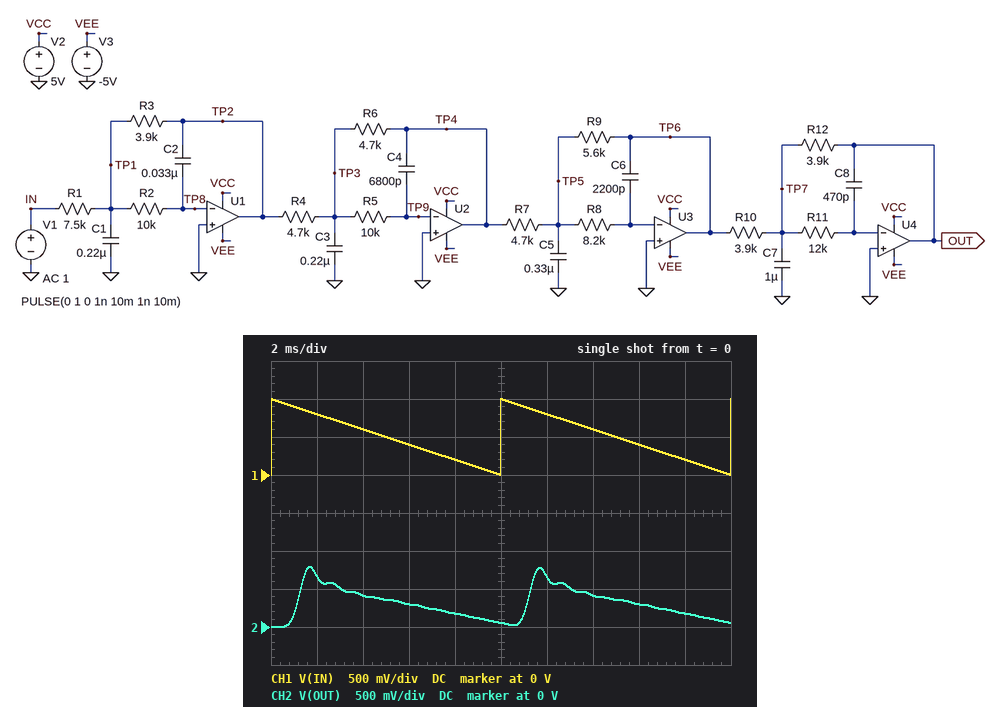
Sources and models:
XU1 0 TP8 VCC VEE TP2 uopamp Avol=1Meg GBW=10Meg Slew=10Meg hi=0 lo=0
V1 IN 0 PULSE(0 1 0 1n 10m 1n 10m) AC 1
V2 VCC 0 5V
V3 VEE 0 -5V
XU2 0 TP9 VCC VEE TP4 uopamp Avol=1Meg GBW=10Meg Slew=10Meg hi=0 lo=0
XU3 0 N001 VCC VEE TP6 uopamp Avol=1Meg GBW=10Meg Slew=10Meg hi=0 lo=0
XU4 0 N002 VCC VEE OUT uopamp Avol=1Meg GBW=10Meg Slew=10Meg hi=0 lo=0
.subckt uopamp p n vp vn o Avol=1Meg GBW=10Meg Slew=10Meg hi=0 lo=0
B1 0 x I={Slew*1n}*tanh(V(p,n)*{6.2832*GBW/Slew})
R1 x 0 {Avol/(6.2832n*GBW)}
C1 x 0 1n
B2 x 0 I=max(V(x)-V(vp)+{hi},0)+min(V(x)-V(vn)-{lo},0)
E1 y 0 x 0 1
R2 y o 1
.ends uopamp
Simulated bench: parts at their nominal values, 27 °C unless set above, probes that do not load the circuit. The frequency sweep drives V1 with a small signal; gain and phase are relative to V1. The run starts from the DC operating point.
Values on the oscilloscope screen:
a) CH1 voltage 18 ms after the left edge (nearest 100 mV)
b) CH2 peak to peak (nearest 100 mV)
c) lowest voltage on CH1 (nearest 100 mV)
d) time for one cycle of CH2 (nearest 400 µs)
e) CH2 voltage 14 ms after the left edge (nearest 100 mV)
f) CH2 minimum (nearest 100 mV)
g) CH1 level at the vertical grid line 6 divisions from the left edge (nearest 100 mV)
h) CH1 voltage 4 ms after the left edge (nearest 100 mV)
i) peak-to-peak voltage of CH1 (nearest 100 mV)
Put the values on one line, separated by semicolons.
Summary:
200 mV; 800 mV; 0 V; 10.0 ms; 400 mV; 0 V; 800 mV; 600 mV; 1.0 V
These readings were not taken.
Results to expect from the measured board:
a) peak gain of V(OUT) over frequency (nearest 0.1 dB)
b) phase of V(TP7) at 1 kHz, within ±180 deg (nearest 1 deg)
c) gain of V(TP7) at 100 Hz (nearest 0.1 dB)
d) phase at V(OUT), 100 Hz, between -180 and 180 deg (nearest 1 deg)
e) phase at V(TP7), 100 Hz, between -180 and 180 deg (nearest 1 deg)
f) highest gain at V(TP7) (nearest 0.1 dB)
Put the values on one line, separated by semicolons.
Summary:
-2.0 dB; 155 deg; -52.5 dB; -33 deg; -123 deg; -35.5 dB
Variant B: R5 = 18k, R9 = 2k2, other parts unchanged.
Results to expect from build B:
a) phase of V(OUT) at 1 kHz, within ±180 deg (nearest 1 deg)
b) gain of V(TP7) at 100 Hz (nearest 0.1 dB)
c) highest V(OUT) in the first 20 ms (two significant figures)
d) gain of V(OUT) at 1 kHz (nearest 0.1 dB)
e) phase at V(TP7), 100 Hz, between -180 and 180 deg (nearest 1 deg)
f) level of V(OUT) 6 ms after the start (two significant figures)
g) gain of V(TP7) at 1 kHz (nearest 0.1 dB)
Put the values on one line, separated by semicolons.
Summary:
-10 deg; -60.6 dB; 280 mV; -23.9 dB; -126 deg; 120 mV; -52.9 dB
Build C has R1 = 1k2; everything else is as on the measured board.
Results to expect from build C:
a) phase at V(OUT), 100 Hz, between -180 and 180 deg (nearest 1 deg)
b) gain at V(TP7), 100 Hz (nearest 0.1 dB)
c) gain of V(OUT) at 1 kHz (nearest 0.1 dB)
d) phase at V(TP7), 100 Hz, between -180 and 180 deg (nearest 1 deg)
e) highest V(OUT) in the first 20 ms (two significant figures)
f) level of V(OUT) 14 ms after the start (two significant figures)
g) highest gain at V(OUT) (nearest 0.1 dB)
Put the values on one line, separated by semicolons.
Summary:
-56 deg; -39.2 dB; 5.7 dB; -146 deg; 3.0 V; 2.7 V; 11.8 dB
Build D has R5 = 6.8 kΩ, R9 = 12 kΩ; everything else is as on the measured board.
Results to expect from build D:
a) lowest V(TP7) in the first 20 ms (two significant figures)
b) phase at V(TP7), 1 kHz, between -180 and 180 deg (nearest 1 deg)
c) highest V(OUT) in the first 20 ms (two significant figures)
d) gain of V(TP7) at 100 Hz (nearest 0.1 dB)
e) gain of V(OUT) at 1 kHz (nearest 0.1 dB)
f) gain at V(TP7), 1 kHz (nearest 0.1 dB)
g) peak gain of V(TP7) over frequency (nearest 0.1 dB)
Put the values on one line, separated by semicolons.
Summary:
-16 mV; 137 deg; 1.9 V; -45.8 dB; -9.1 dB; -38.1 dB; -25.1 dB
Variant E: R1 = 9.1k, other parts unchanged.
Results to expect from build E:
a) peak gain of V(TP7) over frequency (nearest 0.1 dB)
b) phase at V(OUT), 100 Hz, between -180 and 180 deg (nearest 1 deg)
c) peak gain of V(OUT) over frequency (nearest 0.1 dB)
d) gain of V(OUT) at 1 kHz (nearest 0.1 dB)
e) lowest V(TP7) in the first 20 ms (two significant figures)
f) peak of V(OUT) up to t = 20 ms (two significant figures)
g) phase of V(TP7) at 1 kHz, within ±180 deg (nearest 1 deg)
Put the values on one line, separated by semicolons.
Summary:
-37.1 dB; -32 deg; -3.3 dB; -9.7 dB; -6.0 mV; 670 mV; 154 deg
